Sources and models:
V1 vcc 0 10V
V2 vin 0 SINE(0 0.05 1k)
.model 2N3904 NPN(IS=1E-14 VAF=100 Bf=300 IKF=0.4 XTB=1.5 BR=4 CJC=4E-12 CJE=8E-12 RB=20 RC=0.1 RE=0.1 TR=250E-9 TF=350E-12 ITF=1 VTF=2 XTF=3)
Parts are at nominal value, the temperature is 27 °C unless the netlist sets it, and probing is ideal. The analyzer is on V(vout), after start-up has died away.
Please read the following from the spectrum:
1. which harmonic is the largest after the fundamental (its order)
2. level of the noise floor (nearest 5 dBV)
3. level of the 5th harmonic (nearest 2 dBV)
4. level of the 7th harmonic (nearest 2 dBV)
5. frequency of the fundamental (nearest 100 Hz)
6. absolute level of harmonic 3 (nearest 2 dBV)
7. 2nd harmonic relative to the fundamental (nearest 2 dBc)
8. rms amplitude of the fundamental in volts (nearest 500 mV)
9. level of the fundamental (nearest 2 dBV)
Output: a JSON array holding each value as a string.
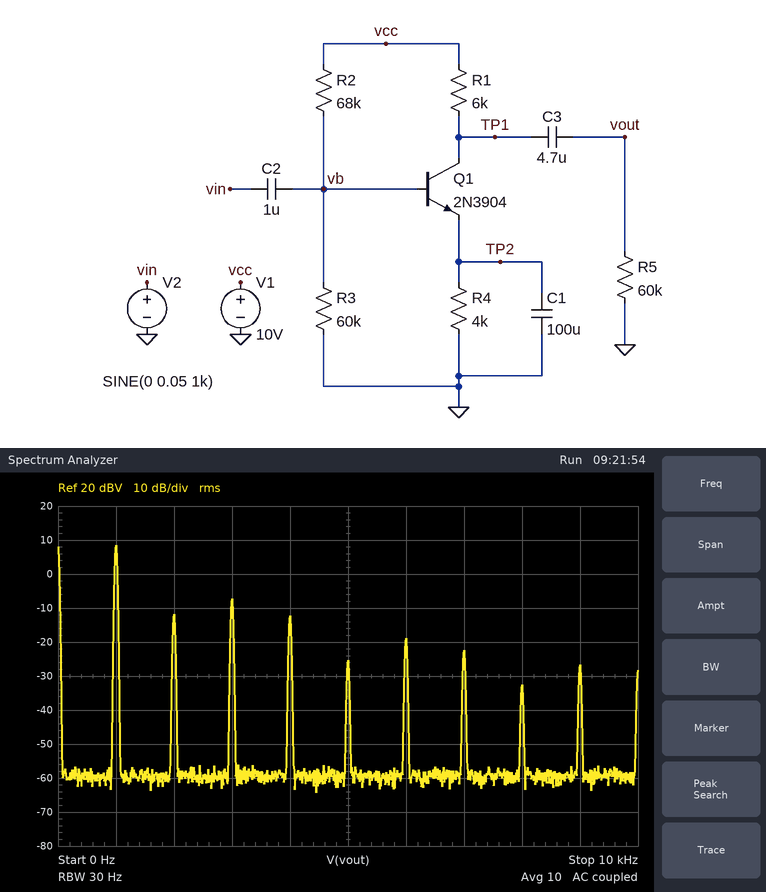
["3", "-60 dBV", "-26 dBV", "-22 dBV", "1.0 kHz", "-8 dBV", "-20 dBc", "2.5 V", "8 dBV"]
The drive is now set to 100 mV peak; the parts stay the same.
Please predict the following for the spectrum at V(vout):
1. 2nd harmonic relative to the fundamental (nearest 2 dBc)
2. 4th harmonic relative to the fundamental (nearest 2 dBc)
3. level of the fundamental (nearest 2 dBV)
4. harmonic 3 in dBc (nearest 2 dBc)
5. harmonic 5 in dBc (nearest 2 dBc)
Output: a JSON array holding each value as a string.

["-8 dBc", "-16 dBc", "10 dBV", "-24 dBc", "-20 dBc"]
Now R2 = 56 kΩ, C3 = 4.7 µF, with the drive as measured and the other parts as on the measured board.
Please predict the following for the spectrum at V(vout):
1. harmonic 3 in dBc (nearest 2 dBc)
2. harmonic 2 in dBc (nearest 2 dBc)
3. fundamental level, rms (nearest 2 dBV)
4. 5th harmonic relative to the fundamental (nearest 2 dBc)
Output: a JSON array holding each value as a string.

["-14 dBc", "-28 dBc", "8 dBV", "-26 dBc"]
